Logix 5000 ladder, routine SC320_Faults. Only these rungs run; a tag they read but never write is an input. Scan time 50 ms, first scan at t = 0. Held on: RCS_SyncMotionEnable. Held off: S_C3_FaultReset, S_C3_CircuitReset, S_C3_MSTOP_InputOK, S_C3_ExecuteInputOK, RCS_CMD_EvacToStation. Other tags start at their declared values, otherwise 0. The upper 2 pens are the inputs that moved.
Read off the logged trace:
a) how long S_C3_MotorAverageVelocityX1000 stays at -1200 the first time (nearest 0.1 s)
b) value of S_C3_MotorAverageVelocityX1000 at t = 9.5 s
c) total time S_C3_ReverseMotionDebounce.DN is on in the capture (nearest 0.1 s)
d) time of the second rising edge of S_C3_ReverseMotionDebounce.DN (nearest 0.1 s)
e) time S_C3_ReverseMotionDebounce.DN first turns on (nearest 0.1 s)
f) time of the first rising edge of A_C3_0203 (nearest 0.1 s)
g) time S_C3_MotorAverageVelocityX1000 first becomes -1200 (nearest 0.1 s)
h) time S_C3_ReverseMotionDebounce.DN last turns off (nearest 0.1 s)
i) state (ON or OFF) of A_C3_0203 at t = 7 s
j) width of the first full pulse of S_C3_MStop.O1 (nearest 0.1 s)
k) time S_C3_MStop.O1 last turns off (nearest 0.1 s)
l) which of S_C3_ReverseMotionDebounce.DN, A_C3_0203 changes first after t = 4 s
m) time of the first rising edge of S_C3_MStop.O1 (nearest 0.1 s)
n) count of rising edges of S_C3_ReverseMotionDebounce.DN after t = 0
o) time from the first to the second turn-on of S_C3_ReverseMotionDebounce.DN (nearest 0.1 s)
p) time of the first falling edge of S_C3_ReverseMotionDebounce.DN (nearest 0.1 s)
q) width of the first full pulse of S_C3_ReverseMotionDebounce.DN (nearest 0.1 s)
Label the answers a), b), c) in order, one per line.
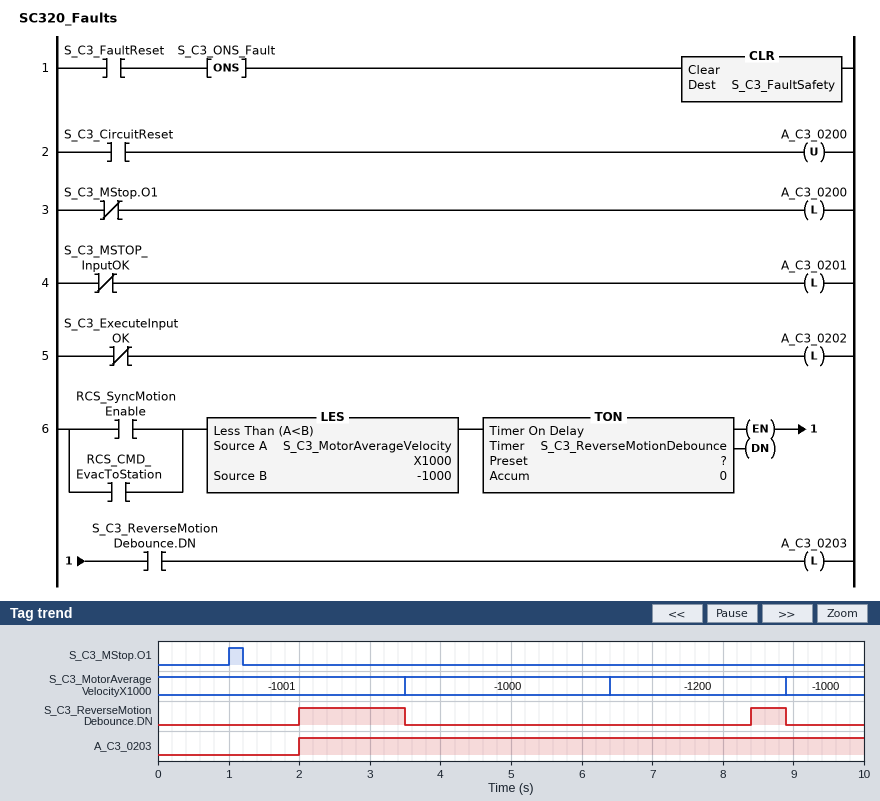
a) 2.5 s
b) -1000
c) 2.0 s
d) 8.4 s
e) 2.0 s
f) 2.0 s
g) 6.4 s
h) 8.9 s
i) ON
j) 0.2 s
k) 1.2 s
l) S_C3_ReverseMotionDebounce.DN
m) 1.0 s
n) 2
o) 6.4 s
p) 3.5 s
q) 1.5 s
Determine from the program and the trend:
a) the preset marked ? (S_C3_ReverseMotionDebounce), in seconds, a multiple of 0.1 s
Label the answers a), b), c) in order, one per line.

a) 2.0 s
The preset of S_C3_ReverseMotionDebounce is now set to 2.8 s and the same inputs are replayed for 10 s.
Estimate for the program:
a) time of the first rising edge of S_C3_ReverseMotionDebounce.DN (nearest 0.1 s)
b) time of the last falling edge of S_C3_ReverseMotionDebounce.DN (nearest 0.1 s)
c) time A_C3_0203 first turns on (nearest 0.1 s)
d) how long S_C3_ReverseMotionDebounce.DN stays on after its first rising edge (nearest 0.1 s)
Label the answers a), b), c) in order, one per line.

a) 2.8 s
b) 3.5 s
c) 2.8 s
d) 0.7 s
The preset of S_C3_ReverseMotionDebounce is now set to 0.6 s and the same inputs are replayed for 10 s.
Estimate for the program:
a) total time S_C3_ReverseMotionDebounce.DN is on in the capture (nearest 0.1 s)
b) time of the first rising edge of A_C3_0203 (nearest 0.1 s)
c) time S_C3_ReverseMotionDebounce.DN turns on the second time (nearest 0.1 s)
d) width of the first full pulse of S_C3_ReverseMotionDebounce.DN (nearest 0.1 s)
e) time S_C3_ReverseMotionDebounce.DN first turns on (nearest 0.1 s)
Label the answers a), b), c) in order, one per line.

a) 4.8 s
b) 0.6 s
c) 7.0 s
d) 2.9 s
e) 0.6 s
